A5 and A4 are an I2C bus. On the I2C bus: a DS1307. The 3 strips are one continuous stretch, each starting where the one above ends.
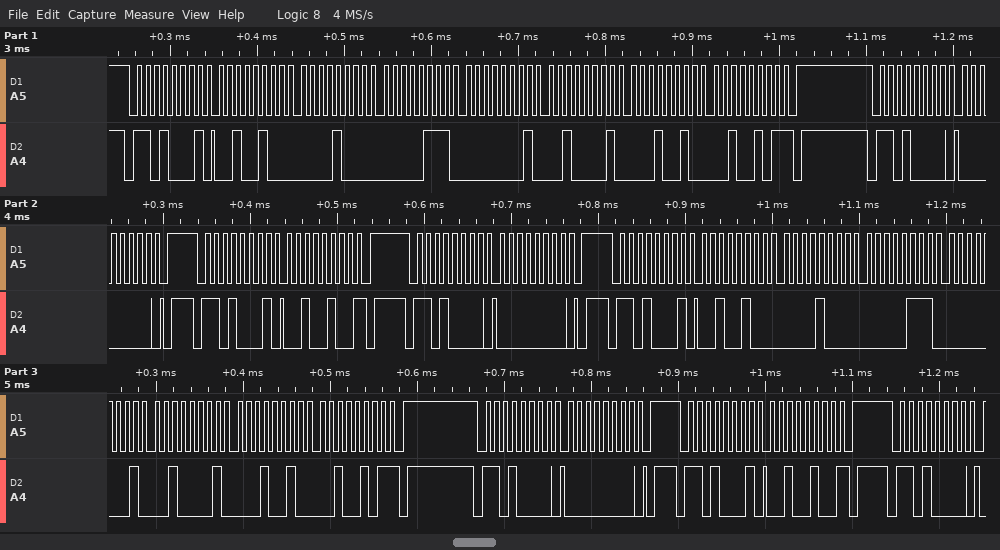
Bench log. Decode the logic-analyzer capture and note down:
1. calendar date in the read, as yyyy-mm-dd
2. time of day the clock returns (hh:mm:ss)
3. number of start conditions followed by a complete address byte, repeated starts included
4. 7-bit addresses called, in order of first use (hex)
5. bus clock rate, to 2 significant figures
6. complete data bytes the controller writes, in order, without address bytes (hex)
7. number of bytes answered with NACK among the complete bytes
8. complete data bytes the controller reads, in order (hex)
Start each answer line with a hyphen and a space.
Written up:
- 2025-12-21
- 07:08:24
- 8
- 0x68
- 100 kHz
- 00 00 00
- 4
- 24 08 07 01 21 12 25 24 24 08 07 01 21 12 25 24
